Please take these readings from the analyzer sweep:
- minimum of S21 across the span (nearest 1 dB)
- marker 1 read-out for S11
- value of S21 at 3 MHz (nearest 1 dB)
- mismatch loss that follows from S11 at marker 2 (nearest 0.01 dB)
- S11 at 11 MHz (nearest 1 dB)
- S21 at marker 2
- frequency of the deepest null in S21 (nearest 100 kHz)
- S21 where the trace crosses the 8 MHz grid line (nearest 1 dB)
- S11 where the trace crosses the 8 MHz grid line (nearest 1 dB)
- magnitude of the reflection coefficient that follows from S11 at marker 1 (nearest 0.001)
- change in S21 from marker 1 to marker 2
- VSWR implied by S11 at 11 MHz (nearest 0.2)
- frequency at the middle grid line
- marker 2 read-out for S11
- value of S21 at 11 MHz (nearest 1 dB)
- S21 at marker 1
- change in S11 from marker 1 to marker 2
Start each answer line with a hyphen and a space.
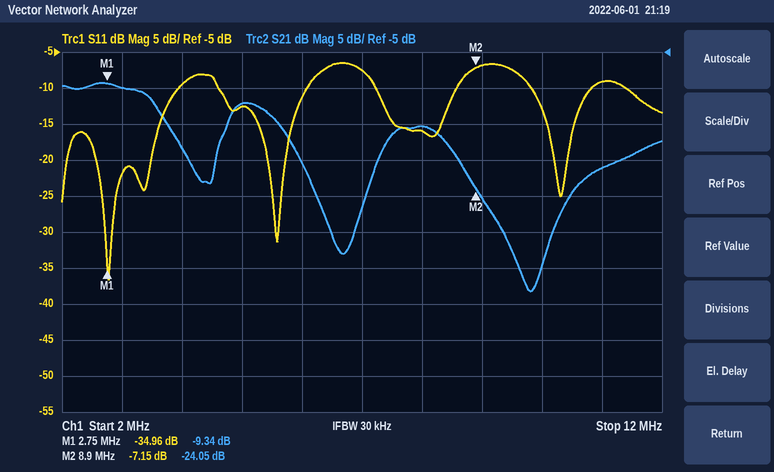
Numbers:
- -38 dB
- -34.96 dB
- -10 dB
- 0.93 dB
- -9 dB
- -24.05 dB
- 9.8 MHz
- -15 dB
- -16 dB
- 0.018
- -14.71 dB
- 2.0
- 7 MHz
- -7.15 dB
- -21 dB
- -9.34 dB
- 27.81 dB
